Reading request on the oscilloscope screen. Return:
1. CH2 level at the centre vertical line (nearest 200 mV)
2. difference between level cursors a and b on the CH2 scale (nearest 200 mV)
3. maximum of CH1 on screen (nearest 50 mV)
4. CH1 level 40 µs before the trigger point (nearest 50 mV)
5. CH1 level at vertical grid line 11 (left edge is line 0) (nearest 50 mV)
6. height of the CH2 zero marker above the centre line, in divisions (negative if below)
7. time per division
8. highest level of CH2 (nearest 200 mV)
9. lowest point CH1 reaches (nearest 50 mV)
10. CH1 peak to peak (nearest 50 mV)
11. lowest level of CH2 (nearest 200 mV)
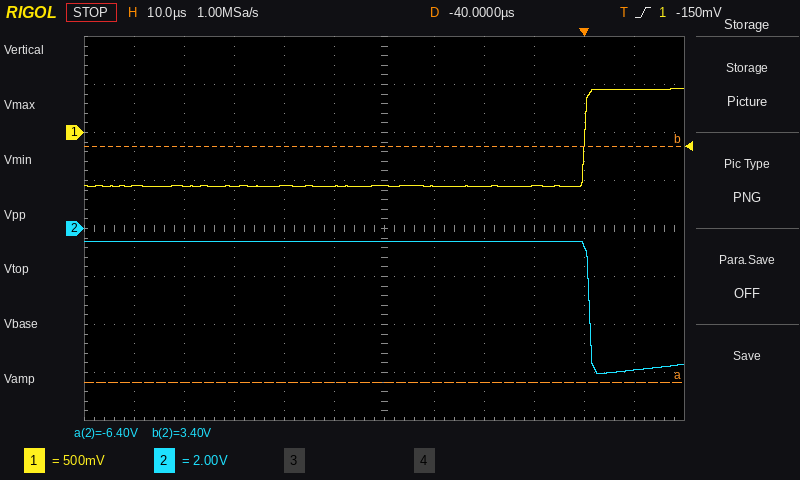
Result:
-600 mV
9.8 V
450 mV
-550 mV
450 mV
0.0 div
10 µs
-600 mV
-550 mV
1.00 V
-6.0 V
